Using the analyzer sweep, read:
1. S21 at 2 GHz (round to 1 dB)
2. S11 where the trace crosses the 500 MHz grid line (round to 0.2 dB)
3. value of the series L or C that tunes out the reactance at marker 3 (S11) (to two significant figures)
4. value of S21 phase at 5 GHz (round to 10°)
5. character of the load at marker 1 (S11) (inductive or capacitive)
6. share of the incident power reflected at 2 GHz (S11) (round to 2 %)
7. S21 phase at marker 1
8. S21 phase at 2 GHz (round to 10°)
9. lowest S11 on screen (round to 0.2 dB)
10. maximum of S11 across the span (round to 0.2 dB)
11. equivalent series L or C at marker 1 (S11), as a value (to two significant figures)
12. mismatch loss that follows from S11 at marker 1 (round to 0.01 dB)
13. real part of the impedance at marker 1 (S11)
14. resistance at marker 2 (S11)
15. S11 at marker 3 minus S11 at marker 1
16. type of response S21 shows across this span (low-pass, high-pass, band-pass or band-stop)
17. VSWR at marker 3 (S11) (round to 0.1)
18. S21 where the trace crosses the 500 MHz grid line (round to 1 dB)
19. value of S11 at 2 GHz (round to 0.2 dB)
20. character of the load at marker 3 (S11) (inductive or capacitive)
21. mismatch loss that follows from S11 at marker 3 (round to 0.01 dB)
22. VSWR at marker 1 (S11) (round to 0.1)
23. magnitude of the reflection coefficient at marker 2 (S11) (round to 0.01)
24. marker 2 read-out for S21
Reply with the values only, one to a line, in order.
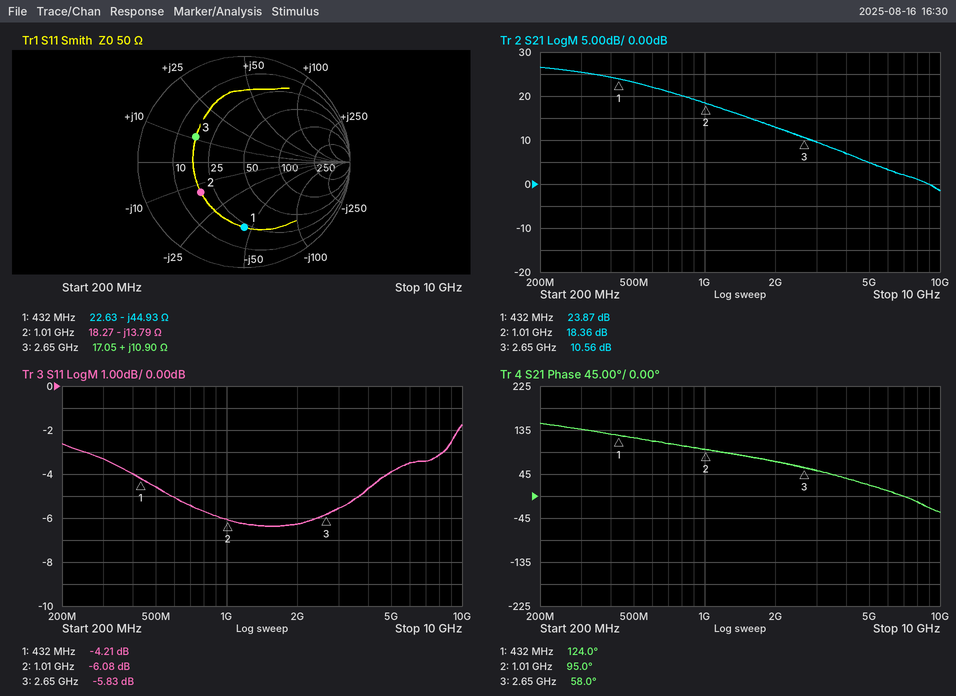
13 dB
-4.6 dB
5.5 pF
20°
capacitive
24 %
124.0°
70°
-6.4 dB
-1.8 dB
8.2 pF
2.07 dB
22.63 Ω
18.27 Ω
-1.62 dB
low-pass
3.1
23 dB
-6.2 dB
inductive
1.31 dB
4.2
0.50
18.36 dB
